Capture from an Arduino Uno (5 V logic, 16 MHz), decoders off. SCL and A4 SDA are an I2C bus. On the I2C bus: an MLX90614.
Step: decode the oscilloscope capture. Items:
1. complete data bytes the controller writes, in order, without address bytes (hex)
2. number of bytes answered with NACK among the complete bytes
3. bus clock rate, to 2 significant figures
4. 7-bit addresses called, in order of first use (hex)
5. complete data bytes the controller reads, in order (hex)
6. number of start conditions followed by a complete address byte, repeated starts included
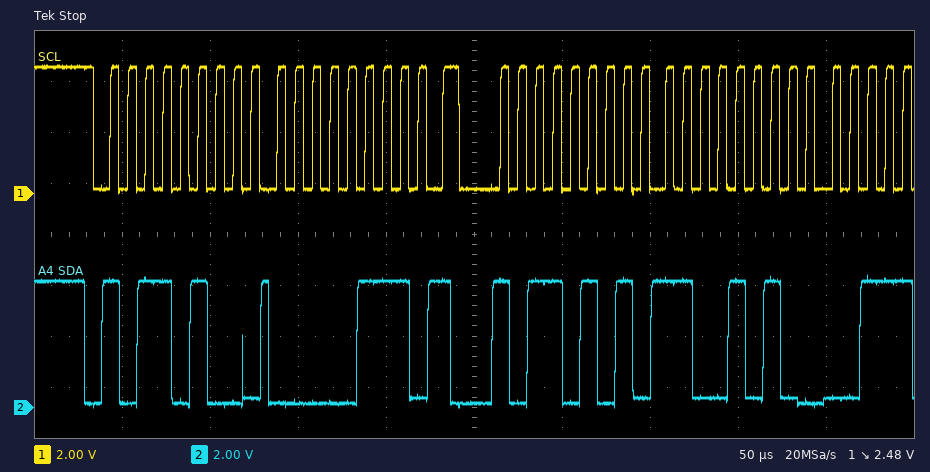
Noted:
07
0
100 kHz
0x5A
CA
2
